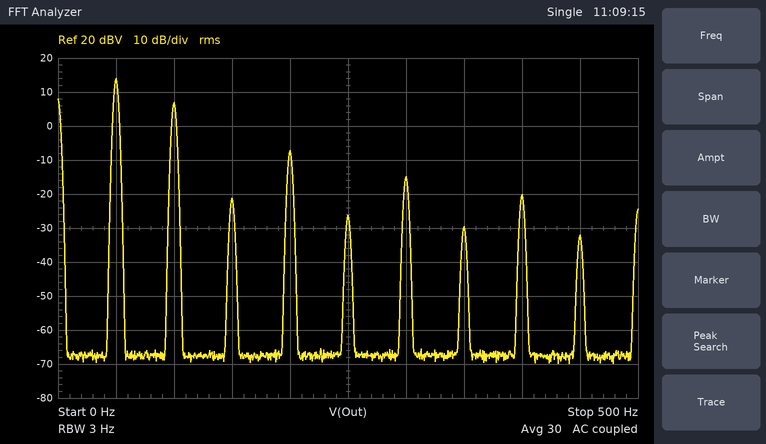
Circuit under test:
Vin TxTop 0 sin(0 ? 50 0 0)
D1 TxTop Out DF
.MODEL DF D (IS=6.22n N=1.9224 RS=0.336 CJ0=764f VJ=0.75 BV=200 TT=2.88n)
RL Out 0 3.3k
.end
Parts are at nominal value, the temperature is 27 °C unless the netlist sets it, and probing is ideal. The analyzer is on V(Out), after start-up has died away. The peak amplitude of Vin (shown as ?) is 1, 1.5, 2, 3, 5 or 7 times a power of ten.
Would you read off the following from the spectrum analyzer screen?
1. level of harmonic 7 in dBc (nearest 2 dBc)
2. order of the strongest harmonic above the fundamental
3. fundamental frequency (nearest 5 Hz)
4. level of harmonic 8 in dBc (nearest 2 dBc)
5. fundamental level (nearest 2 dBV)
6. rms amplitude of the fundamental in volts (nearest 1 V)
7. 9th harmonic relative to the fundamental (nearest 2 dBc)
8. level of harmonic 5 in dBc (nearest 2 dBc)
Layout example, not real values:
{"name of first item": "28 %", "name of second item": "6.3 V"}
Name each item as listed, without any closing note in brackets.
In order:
{"level of harmonic 7 in dBc": "-44 dBc", "order of the strongest harmonic above the fundamental": "2", "fundamental frequency": "50 Hz", "level of harmonic 8 in dBc": "-34 dBc", "fundamental level": "14 dBV", "rms amplitude of the fundamental in volts": "5 V", "9th harmonic relative to the fundamental": "-46 dBc", "level of harmonic 5 in dBc": "-40 dBc"}
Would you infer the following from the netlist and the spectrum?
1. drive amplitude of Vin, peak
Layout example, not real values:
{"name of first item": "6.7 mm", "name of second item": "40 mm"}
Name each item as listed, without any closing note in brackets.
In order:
{"drive amplitude of Vin, peak": "15 V"}
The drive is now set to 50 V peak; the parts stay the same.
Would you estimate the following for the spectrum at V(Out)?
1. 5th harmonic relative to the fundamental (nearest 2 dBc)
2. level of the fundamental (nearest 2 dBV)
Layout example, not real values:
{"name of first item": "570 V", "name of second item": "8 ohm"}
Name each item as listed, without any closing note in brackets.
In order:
{"5th harmonic relative to the fundamental": "-50 dBc", "level of the fundamental": "24 dBV"}
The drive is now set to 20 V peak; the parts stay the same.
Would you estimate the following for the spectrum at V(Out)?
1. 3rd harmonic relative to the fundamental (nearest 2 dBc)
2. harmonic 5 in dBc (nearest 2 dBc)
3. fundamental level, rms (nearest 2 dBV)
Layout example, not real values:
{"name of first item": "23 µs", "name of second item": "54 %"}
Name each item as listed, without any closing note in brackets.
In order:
{"3rd harmonic relative to the fundamental": "-38 dBc", "harmonic 5 in dBc": "-42 dBc", "fundamental level, rms": "16 dBV"}
